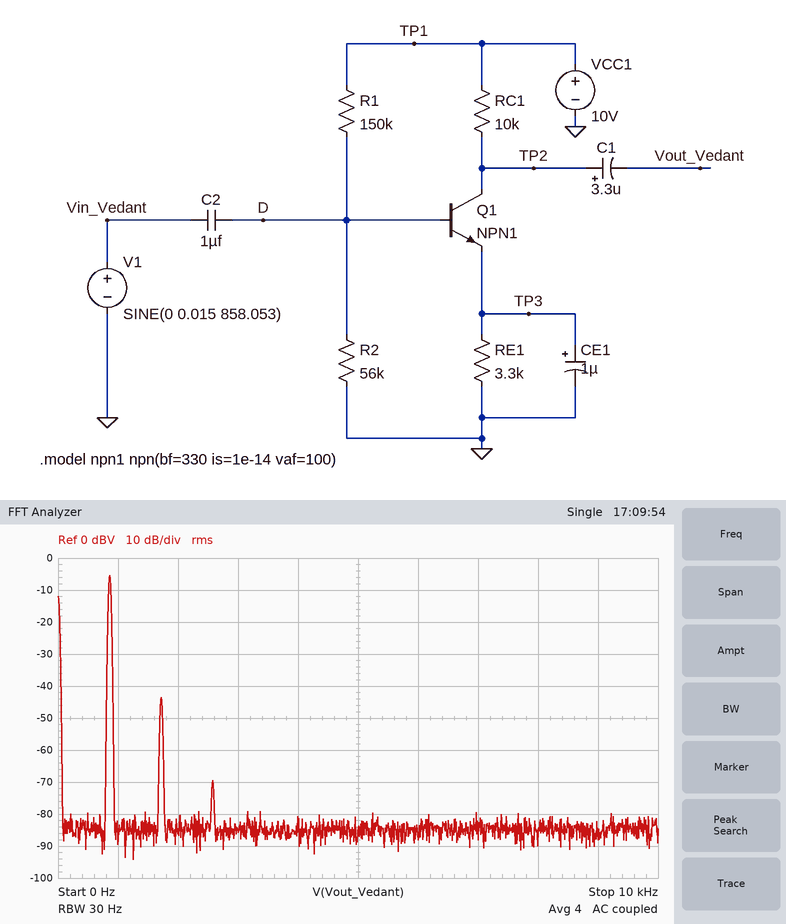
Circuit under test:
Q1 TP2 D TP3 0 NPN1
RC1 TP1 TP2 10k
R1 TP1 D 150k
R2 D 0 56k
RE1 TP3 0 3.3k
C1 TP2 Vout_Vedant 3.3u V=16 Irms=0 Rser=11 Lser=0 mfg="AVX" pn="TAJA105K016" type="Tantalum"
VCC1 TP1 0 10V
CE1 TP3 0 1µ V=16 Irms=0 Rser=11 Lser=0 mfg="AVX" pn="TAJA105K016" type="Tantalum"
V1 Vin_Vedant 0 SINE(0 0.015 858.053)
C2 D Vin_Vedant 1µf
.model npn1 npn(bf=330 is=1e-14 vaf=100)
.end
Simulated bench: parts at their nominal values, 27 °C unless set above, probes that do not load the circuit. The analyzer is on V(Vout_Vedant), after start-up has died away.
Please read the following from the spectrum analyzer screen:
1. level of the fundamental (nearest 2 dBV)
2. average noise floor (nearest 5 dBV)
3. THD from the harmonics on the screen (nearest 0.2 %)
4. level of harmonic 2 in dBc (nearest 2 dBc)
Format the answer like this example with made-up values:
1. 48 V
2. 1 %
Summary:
1. -6 dBV
2. -85 dBV
3. 1.2 %
4. -38 dBc
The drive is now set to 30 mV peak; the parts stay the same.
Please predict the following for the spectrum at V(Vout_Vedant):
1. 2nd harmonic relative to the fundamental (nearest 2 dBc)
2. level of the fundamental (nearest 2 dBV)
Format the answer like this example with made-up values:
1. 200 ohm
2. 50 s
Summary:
1. -32 dBc
2. 0 dBV
